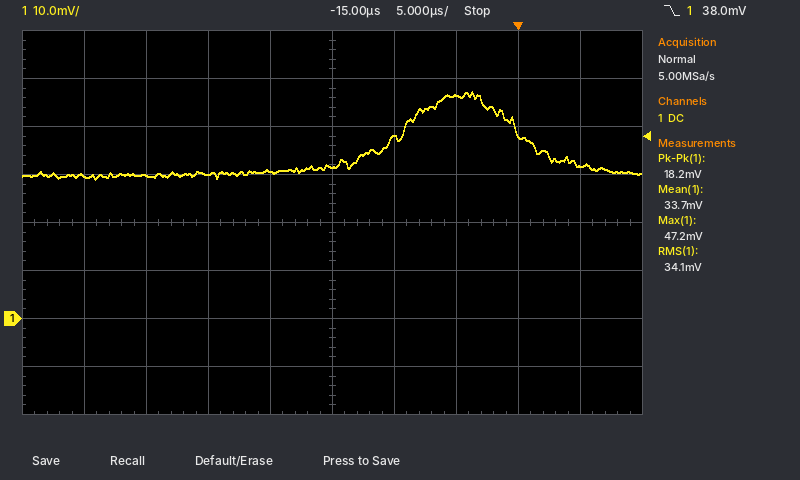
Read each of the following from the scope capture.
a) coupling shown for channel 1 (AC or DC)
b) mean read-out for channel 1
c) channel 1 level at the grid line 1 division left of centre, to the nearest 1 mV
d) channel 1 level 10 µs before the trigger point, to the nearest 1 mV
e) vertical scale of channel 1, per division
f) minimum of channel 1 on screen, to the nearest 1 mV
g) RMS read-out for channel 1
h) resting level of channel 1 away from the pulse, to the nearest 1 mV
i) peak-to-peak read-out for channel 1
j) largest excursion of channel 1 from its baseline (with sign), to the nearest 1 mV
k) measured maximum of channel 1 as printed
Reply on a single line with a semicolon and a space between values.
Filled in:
DC; 33.7 mV; 31 mV; 38 mV; 10 mV; 29 mV; 34.1 mV; 30 mV; 18.2 mV; +17 mV; 47.2 mV
